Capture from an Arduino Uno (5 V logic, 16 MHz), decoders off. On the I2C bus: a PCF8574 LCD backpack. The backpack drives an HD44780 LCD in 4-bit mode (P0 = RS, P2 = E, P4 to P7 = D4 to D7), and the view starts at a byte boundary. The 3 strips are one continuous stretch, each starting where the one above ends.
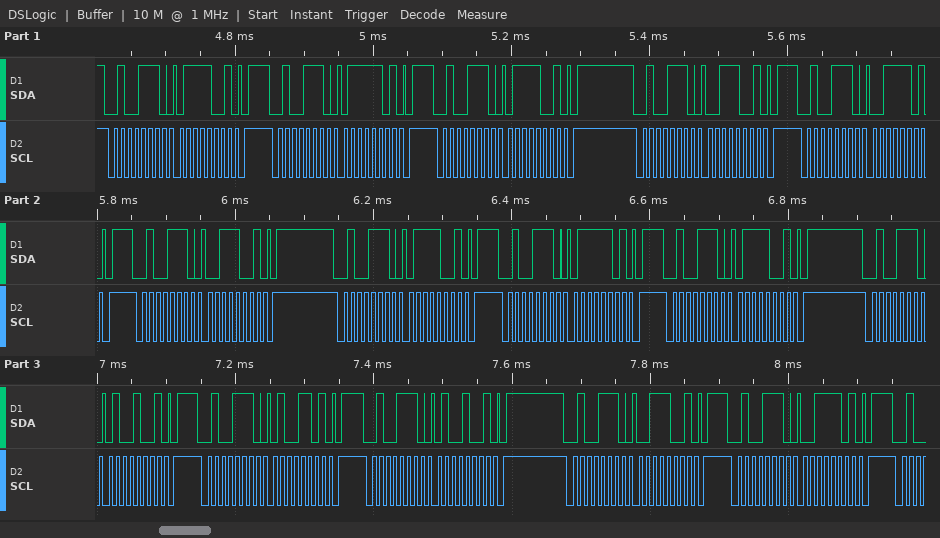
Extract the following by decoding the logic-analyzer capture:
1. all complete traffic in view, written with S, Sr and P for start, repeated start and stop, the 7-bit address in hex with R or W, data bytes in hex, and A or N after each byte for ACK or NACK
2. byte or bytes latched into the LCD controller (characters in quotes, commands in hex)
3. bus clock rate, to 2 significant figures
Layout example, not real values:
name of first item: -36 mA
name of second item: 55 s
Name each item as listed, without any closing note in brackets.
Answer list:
all complete traffic in view, written with S, Sr and P for start, repeated start and stop, the 7-bit address in hex with R or W, data bytes in hex, and A or N after each byte for ACK or NACK: S 27W A 79 A P S 27W A 7D A P S 27W A 79 A P S 27W A 39 A P S 27W A 3D A P S 27W A 39 A P S 27W A 79 A P S 27W A 7D A P S 27W A 79 A P S 27W A 49 A P S 27W A 4D A P S 27W A 49 A P S 27W A 39 A P S 27W A 3D A P
byte or bytes latched into the LCD controller: 's' 't'
bus clock rate, to 2 significant figures: 100 kHz
